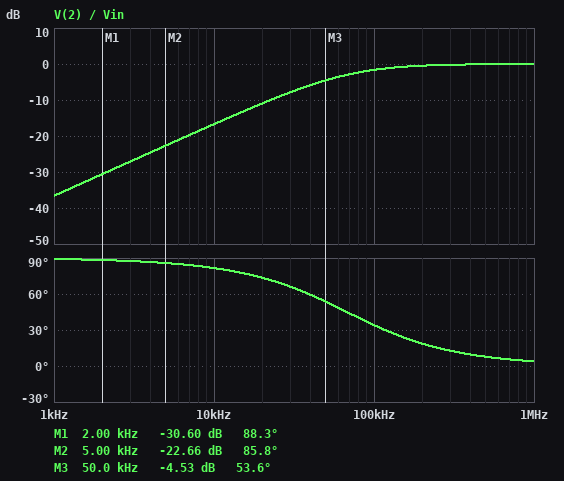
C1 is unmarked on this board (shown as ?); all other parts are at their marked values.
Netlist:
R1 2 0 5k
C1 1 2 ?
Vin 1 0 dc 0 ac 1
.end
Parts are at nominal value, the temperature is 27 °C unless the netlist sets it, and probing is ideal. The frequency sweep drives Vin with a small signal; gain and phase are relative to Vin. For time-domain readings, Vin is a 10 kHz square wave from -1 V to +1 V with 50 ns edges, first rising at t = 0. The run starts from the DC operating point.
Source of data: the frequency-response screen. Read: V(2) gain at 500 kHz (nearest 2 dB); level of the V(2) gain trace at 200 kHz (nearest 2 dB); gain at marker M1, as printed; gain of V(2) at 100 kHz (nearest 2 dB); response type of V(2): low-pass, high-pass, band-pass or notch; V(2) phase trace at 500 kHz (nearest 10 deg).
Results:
0 dB
0 dB
-30.60 dB
-2 dB
high-pass
10 deg
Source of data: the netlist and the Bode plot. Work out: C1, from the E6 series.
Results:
470 pF
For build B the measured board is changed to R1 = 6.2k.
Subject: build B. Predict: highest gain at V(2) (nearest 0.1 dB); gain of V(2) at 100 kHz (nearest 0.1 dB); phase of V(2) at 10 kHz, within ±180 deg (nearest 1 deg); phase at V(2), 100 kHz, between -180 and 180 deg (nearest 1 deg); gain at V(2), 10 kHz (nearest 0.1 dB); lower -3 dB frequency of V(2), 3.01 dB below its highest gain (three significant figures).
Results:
0 dB
-1.1 dB
80 deg
29 deg
-14.9 dB
54.6 kHz
